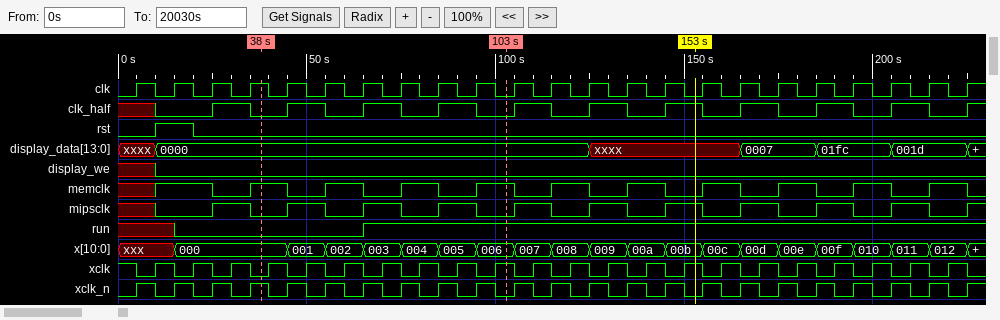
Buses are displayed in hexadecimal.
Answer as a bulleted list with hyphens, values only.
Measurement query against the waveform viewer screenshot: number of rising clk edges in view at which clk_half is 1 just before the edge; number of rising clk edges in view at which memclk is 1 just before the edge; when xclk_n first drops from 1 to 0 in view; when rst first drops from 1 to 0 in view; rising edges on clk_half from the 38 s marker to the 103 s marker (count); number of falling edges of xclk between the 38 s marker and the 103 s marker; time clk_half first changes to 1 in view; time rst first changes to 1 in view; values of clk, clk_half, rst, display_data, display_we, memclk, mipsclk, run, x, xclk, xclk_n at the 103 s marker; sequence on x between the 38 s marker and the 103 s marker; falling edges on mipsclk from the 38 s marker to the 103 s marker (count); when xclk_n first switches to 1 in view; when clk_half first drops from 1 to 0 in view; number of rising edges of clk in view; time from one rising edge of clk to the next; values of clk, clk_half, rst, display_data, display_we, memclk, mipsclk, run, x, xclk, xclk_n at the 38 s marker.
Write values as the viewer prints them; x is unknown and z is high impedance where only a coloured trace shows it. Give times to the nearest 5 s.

- 10
- 12
- 10 s
- 20 s
- 3
- 6
- 25 s
- 10 s
- clk=0, clk_half=0, rst=0, display_data=0000, display_we=0, memclk=1, mipsclk=0, run=1, x=006, xclk=1, xclk_n=0
- 000, 001, 002, 003, 004, 005, 006
- 3
- 5 s
- 35 s
- 23
- 10 s
- clk=1, clk_half=0, rst=0, display_data=0000, display_we=0, memclk=1, mipsclk=0, run=0, x=000, xclk=0, xclk_n=1
